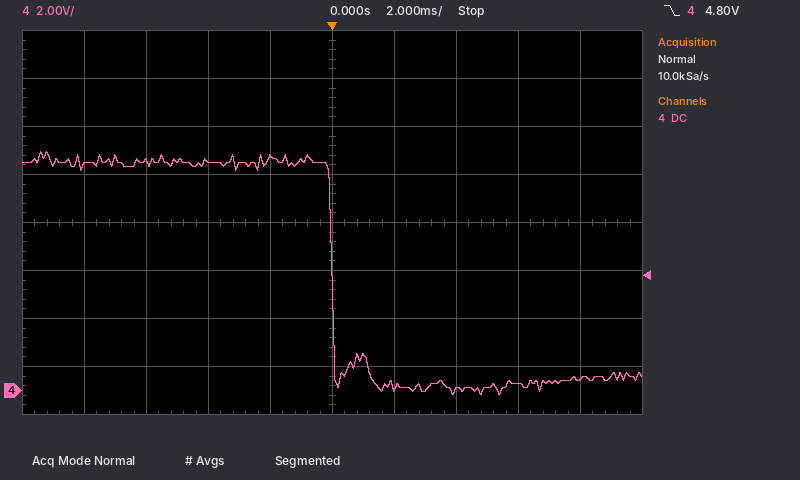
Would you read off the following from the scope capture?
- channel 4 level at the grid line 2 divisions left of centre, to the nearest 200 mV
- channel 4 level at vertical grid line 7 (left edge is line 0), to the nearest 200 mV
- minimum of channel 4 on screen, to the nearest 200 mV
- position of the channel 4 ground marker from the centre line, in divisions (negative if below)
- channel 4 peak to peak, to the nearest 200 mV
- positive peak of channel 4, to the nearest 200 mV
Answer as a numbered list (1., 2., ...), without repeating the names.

1. 9.6 V
2. 0.0 V
3. -200 mV
4. -3.5 div
5. 10.2 V
6. 10.0 V
